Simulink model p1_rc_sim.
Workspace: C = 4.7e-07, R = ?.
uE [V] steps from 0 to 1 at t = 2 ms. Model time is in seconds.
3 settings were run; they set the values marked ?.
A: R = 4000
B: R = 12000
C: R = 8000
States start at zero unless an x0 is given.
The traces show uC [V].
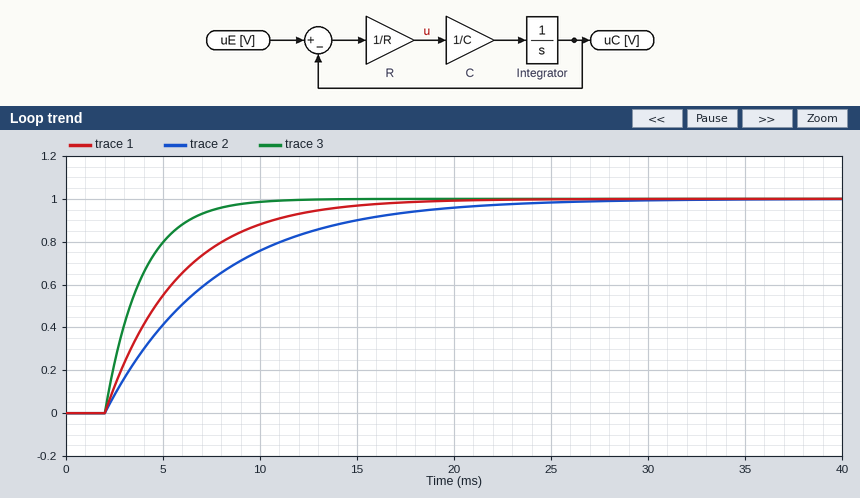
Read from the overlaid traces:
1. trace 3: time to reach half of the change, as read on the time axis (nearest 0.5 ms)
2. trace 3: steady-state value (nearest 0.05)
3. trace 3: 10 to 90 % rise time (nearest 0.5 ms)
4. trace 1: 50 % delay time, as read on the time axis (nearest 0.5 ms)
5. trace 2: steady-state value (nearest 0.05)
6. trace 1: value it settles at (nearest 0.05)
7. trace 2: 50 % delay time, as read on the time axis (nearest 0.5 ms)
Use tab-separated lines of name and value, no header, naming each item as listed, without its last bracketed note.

trace 3: time to reach half of the change, as read on the time axis	3.5 ms
trace 3: steady-state value	1.00
trace 3: 10 to 90 % rise time	4.0 ms
trace 1: 50 % delay time, as read on the time axis	4.5 ms
trace 2: steady-state value	1.00
trace 1: value it settles at	1.00
trace 2: 50 % delay time, as read on the time axis	6.0 ms
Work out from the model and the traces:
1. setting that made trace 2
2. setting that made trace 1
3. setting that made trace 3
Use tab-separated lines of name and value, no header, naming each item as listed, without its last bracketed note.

setting that made trace 2	B
setting that made trace 1	C
setting that made trace 3	A
